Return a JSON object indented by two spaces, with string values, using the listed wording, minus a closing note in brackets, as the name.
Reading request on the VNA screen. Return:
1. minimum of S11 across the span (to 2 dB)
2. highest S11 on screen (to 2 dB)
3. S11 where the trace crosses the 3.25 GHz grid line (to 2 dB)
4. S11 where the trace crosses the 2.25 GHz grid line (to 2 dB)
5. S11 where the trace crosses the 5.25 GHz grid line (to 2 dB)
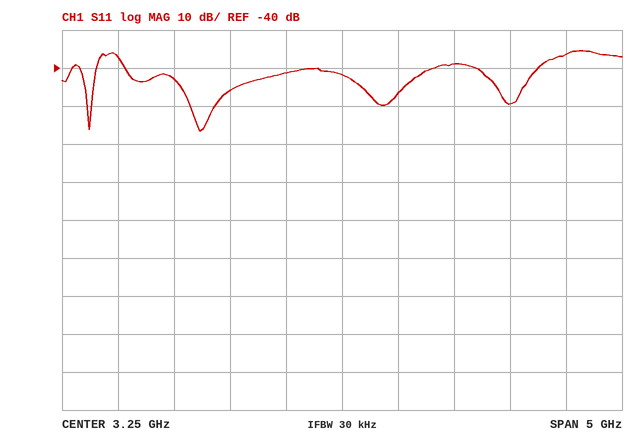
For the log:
{
  "minimum of S11 across the span": "-56 dB",
  "highest S11 on screen": "-36 dB",
  "S11 where the trace crosses the 3.25 GHz grid line": "-42 dB",
  "S11 where the trace crosses the 2.25 GHz grid line": "-46 dB",
  "S11 where the trace crosses the 5.25 GHz grid line": "-36 dB"
}
